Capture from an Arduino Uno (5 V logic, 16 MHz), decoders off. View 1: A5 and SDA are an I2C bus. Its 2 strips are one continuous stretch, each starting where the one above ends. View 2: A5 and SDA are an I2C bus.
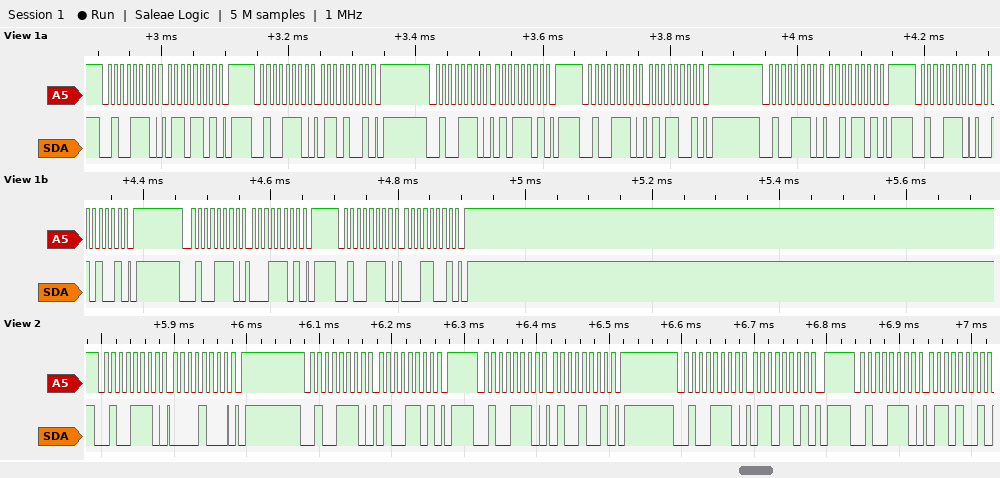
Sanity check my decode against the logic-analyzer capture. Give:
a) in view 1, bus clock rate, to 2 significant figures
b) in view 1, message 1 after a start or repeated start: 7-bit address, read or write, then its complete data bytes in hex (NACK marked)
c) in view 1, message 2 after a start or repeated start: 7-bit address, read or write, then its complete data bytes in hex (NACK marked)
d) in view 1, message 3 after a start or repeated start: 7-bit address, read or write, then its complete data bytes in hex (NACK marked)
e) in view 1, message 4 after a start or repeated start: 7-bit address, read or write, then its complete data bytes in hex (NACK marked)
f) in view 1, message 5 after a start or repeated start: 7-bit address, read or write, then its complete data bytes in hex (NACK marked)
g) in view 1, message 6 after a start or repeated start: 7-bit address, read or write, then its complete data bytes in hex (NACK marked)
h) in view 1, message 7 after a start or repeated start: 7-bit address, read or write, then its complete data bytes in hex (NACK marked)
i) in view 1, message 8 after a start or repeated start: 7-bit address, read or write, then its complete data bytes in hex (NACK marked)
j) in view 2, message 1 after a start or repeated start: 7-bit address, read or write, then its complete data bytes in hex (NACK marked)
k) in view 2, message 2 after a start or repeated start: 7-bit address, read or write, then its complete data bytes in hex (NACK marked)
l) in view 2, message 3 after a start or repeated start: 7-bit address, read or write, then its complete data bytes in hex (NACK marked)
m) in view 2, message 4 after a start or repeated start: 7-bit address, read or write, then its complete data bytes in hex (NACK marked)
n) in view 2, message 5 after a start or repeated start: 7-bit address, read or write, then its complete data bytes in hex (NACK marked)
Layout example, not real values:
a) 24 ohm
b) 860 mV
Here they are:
a) 100 kHz
b) 0x27 write: 6D
c) 0x27 write: 69
d) 0x27 write: 5D
e) 0x27 write: 59
f) 0x27 write: 2D
g) 0x27 write: 29
h) 0x27 write: 1D
i) 0x27 write: 19
j) 0x27 write: 08
k) 0x27 write: 4D
l) 0x27 write: 49
m) 0x27 write: 6D
n) 0x27 write: 69
